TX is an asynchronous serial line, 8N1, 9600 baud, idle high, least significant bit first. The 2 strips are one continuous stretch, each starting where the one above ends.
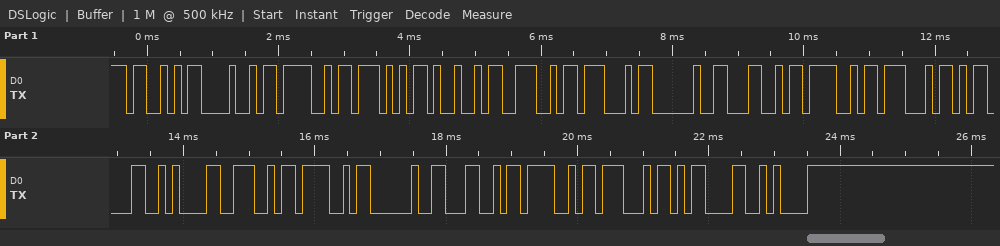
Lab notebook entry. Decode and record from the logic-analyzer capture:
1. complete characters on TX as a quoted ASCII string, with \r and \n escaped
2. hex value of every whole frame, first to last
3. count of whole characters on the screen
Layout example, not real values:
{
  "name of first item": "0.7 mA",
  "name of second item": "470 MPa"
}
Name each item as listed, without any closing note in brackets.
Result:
{
  "complete characters on TX as a quoted ASCII string, with \\r and \\n escaped": "\"SHOWING LOG\\r\\nNO LOG\\r\\n\"",
  "hex value of every whole frame, first to last": "53 48 4F 57 49 4E 47 20 4C 4F 47 0D 0A 4E 4F 20 4C 4F 47 0D 0A",
  "count of whole characters on the screen": "21"
}
